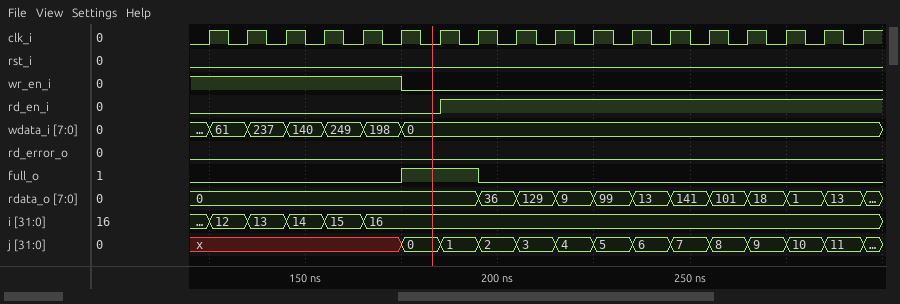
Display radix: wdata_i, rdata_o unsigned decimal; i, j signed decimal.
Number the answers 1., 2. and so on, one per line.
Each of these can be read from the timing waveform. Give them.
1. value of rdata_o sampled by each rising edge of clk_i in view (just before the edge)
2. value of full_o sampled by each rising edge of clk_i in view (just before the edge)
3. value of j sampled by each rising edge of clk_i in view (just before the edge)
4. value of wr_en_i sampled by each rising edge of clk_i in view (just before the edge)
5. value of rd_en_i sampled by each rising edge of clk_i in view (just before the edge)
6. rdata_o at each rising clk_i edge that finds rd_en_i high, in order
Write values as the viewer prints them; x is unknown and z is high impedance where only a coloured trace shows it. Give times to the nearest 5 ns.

1. 0, 0, 0, 0, 0, 0, 0, 0, 36, 129, 9, 99, 13, 141, 101, 18, 1, 13
2. 0 0 0 0 0 0 1 1 0 0 0 0 0 0 0 0 0 0
3. x, x, x, x, x, x, 0, 1, 2, 3, 4, 5, 6, 7, 8, 9, 10, 11
4. 1 1 1 1 1 1 0 0 0 0 0 0 0 0 0 0 0 0
5. 0 0 0 0 0 0 0 1 1 1 1 1 1 1 1 1 1 1
6. 0, 36, 129, 9, 99, 13, 141, 101, 18, 1, 13
